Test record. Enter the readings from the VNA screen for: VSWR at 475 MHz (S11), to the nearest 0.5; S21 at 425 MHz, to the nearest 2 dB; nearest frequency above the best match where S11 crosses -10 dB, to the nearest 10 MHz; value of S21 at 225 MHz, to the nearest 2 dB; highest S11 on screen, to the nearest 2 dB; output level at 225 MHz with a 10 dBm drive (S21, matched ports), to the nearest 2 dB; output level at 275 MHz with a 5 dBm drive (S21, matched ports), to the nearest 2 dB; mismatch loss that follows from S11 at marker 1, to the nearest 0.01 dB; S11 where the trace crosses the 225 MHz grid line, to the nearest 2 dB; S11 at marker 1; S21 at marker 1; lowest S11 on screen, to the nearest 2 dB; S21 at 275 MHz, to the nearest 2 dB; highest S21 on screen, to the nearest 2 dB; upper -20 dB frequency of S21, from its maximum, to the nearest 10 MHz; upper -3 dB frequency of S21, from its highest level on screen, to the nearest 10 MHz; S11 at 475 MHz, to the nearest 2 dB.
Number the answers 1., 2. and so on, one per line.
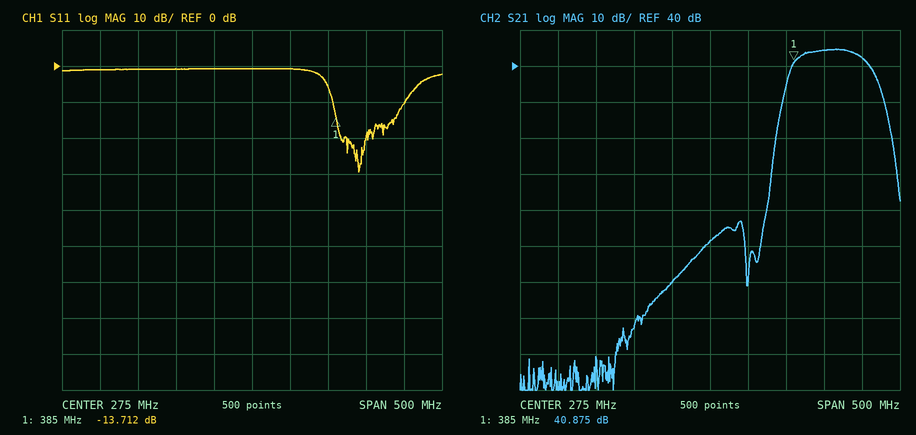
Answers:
1. 2.0
2. 44 dB
3. 480 MHz
4. -20 dB
5. 0 dB
6. -10 dBm
7. -4 dBm
8. 0.19 dB
9. 0 dB
10. -13.712 dB
11. 40.875 dB
12. -30 dB
13. -8 dB
14. 44 dB
15. 510 MHz
16. 480 MHz
17. -10 dB
